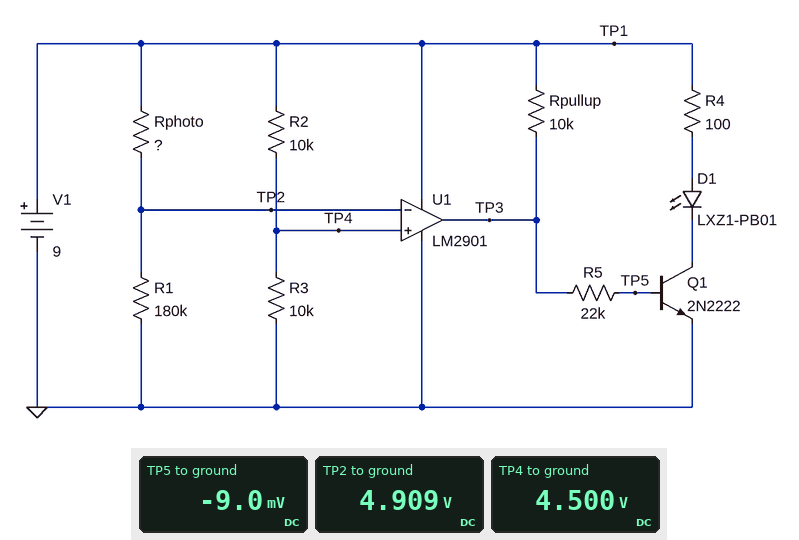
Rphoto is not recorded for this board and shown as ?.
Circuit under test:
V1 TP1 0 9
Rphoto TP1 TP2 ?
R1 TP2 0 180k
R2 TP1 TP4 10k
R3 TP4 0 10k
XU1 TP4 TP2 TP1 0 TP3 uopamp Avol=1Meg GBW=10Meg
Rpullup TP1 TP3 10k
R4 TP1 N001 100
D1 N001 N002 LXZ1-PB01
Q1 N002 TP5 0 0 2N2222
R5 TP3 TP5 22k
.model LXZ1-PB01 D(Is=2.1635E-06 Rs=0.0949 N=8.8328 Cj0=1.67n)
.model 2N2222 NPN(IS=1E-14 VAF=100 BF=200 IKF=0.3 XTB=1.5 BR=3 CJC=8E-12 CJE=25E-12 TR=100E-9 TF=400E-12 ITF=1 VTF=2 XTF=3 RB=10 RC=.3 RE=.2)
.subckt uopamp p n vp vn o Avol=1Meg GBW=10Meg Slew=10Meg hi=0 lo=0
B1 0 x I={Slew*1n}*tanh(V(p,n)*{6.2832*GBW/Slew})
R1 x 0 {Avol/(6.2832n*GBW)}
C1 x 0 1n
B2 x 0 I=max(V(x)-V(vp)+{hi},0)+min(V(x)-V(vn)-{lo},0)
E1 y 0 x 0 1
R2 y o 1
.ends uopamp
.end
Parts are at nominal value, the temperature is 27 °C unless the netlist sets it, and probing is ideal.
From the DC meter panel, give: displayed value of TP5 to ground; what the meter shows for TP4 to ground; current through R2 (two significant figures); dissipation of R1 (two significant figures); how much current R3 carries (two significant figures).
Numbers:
-9.0 mV
4.500 V
450 µA
130 µW
450 µA
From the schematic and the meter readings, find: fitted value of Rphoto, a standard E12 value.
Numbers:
150 kΩ
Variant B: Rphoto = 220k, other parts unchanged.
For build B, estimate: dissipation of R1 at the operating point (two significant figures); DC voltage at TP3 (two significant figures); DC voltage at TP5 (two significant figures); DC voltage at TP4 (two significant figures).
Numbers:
91 µW
9.0 V
780 mV
4.5 V
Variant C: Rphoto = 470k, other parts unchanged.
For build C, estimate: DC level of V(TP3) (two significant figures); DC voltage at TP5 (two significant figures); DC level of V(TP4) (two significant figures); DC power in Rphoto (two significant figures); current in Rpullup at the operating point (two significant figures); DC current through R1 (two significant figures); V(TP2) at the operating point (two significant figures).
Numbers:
9.0 V
780 mV
4.5 V
90 µW
960 nA
14 µA
2.5 V
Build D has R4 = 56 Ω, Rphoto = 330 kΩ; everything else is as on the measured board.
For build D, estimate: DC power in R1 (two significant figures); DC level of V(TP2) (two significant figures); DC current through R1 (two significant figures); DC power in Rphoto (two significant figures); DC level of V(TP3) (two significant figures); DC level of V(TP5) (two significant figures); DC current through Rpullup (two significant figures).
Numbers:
56 µW
3.2 V
18 µA
100 µW
9.0 V
780 mV
960 nA
